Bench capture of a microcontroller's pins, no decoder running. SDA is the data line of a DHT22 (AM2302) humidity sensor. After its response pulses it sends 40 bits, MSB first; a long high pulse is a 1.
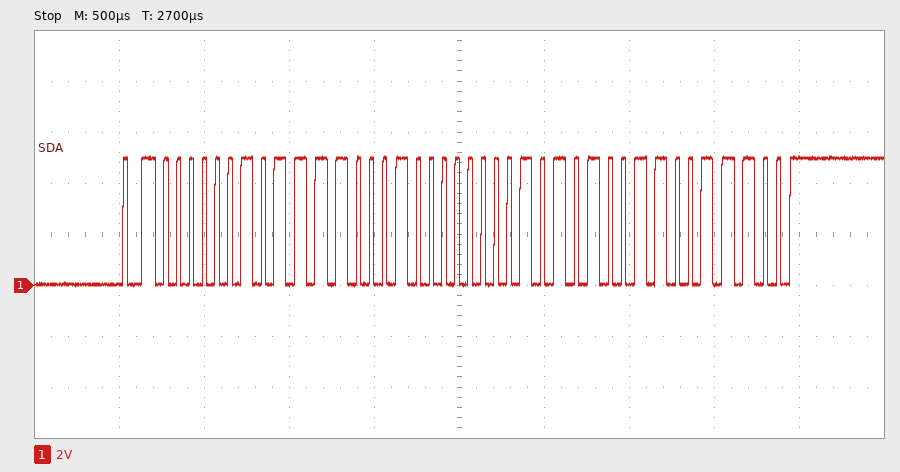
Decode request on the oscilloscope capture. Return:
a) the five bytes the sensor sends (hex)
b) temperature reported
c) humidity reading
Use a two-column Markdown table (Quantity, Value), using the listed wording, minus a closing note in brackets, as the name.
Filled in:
| Quantity | Value |
|---|---|
| the five bytes the sensor sends | 02 F1 00 A9 9C |
| temperature reported | 16.9 °C |
| humidity reading | 75.3 % |
